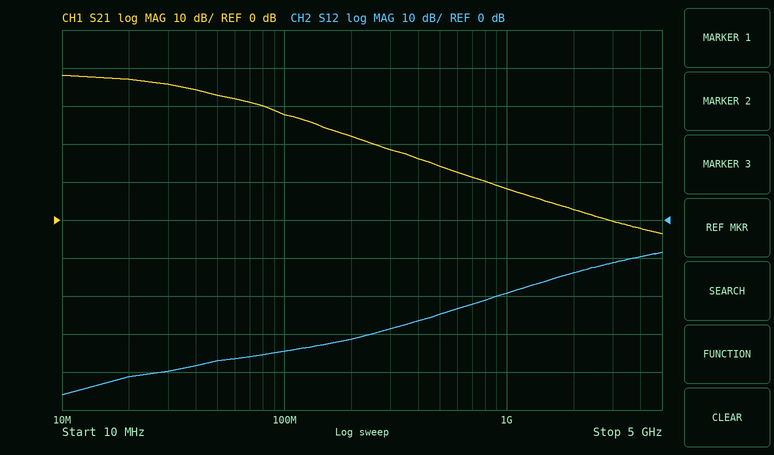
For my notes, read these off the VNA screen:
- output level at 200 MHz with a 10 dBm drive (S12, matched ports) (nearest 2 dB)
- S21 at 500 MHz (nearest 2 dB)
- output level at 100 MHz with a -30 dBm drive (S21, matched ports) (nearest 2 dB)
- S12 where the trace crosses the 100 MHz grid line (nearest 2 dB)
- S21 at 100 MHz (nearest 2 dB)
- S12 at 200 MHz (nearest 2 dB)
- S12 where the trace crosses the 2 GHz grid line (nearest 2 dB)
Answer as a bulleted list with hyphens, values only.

- -22 dBm
- 14 dB
- -2 dBm
- -34 dB
- 28 dB
- -32 dB
- -14 dB
